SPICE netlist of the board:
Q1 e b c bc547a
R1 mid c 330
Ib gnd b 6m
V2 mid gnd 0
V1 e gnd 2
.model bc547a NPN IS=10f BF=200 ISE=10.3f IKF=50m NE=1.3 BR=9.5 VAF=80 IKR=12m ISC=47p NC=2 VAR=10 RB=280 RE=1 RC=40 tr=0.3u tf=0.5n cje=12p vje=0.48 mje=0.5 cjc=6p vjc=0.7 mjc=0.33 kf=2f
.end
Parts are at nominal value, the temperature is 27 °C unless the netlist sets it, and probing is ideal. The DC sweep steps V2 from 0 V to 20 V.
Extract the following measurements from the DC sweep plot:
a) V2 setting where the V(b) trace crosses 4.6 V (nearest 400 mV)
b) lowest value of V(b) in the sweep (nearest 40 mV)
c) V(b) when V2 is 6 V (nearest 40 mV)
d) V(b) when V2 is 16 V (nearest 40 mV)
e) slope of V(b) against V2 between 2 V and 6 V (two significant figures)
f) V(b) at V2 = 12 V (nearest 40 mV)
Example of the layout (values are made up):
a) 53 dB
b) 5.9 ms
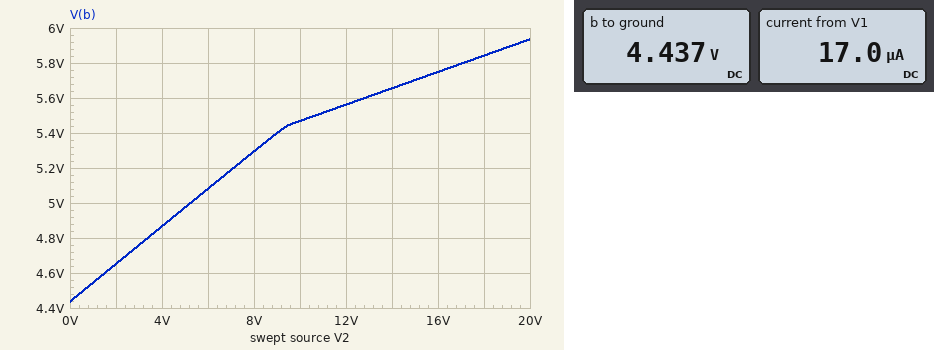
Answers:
a) 1.6 V
b) 4.44 V
c) 5.08 V
d) 5.76 V
e) 0.11 V/V
f) 5.56 V
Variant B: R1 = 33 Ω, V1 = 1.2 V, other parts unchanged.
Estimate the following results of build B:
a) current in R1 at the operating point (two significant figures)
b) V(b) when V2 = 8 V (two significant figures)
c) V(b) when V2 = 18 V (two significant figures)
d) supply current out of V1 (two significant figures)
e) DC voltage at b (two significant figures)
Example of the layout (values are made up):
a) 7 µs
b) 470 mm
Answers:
a) 19 mA
b) 5.0 V
c) 5.7 V
d) 13 mA
e) 3.1 V
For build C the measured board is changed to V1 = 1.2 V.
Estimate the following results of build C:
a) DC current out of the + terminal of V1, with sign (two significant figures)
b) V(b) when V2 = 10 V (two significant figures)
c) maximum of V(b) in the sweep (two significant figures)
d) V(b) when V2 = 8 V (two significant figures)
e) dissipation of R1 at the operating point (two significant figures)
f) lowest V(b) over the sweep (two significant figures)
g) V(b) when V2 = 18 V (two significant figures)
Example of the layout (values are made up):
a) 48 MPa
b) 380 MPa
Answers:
a) -2.1 mA
b) 4.7 V
c) 5.2 V
d) 4.6 V
e) 4.9 mW
f) 3.7 V
g) 5.1 V
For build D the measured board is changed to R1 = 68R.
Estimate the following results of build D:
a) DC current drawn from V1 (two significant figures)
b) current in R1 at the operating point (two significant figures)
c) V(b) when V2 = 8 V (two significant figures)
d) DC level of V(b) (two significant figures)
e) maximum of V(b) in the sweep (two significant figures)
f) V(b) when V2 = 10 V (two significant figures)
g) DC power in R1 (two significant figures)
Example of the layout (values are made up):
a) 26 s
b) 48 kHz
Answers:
a) 14 mA
b) 20 mA
c) 5.7 V
d) 3.9 V
e) 6.5 V
f) 5.8 V
g) 28 mW
